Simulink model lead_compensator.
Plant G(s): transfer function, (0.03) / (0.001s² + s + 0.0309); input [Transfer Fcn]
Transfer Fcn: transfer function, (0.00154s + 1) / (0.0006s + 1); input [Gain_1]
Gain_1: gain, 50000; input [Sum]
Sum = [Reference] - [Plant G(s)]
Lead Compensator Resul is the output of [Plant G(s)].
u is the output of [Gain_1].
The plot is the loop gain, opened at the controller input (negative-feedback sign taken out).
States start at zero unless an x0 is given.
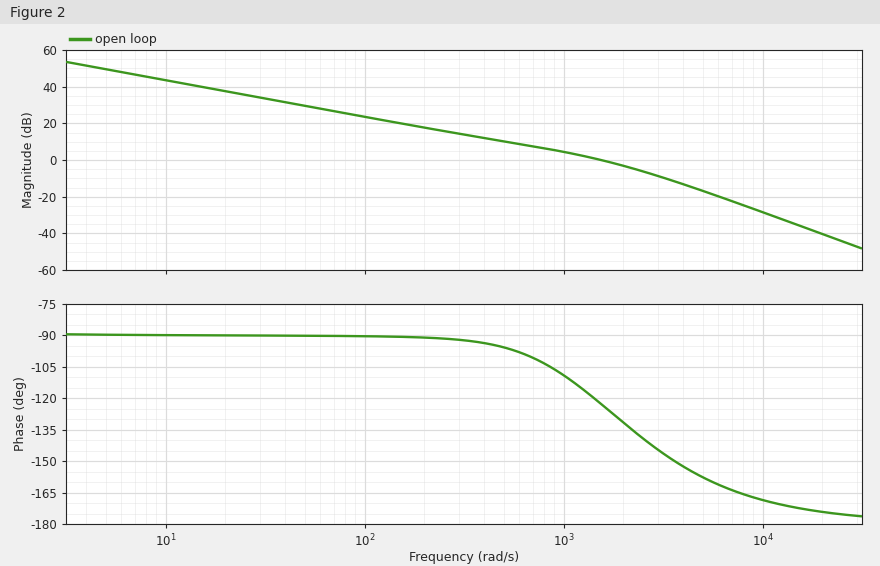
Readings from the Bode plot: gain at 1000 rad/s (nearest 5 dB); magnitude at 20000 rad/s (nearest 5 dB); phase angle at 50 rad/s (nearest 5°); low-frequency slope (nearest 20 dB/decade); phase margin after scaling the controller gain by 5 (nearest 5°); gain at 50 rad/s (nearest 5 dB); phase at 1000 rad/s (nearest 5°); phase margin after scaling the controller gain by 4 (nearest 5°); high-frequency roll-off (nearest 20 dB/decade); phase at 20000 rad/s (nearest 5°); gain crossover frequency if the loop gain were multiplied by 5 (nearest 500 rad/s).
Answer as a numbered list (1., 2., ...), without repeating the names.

1. 5 dB
2. -40 dB
3. -90°
4. -20 dB/decade
5. 25°
6. 30 dB
7. -110°
8. 30°
9. -40 dB/decade
10. -175°
11. 4000 rad/s
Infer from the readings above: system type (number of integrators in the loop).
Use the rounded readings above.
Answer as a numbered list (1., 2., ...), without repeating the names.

1. 1
